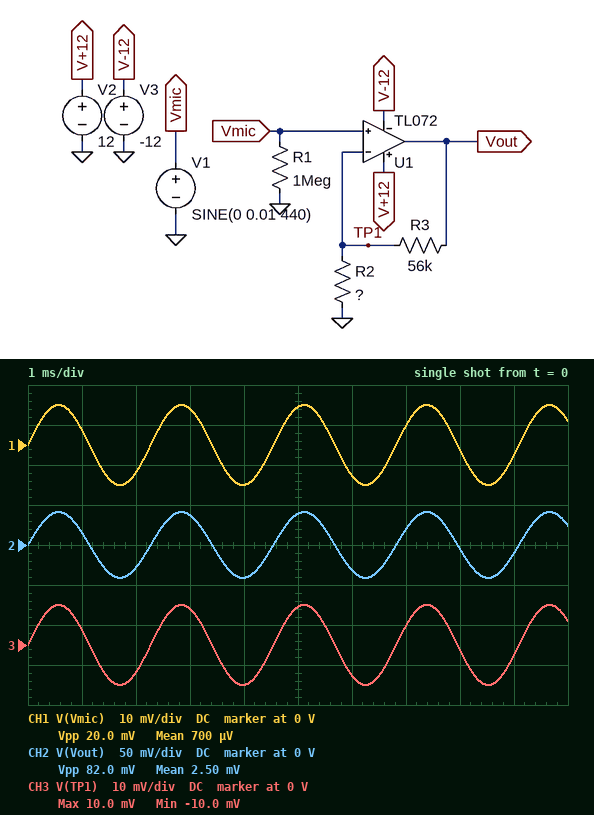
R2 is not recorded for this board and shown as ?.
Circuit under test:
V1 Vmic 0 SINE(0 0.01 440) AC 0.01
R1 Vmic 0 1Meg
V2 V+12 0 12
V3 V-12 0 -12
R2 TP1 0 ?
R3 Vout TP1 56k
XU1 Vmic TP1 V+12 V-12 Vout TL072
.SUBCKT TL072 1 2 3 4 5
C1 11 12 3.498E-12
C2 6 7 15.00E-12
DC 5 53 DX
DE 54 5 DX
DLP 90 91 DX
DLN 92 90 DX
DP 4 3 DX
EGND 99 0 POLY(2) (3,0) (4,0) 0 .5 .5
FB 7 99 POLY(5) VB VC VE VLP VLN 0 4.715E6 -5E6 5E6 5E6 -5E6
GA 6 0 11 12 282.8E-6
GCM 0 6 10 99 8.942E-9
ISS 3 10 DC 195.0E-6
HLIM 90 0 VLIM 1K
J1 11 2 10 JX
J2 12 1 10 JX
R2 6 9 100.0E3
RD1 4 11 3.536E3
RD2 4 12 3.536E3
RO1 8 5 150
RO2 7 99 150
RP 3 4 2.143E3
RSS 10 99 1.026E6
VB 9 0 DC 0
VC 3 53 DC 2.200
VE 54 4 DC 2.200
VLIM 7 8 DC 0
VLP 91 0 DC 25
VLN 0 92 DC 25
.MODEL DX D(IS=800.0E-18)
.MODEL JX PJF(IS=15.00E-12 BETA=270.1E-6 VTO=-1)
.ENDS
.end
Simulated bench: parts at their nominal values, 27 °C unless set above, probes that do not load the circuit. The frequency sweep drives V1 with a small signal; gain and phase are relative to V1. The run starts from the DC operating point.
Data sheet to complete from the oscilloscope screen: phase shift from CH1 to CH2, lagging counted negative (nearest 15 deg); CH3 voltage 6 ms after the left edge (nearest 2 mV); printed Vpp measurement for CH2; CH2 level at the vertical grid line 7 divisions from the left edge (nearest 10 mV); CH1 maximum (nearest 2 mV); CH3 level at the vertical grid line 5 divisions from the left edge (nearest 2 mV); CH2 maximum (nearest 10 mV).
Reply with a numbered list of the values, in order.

1. 0 deg
2. -8 mV
3. 82.0 mV
4. 20 mV
5. 10 mV
6. 10 mV
7. 40 mV
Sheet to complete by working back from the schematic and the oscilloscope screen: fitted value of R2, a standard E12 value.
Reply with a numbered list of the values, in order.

1. 18 kΩ
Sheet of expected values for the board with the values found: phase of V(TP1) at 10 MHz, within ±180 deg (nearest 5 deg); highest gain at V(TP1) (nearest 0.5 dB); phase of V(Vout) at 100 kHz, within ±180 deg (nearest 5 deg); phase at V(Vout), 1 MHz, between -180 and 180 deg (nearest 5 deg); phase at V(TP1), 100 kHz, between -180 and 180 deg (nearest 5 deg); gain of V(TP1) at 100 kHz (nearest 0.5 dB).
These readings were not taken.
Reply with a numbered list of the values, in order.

1. -145 deg
2. 0 dB
3. -5 deg
4. -55 deg
5. -5 deg
6. 0 dB
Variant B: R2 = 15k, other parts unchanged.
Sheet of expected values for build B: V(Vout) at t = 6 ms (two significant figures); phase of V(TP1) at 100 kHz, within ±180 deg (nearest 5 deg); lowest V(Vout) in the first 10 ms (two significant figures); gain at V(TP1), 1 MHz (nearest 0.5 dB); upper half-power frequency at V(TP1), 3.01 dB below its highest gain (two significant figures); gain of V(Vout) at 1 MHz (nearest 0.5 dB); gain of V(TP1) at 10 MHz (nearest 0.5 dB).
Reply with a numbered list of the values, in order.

1. -36 mV
2. -10 deg
3. -47 mV
4. -4.0 dB
5. 820 kHz
6. 9.5 dB
7. -28.0 dB
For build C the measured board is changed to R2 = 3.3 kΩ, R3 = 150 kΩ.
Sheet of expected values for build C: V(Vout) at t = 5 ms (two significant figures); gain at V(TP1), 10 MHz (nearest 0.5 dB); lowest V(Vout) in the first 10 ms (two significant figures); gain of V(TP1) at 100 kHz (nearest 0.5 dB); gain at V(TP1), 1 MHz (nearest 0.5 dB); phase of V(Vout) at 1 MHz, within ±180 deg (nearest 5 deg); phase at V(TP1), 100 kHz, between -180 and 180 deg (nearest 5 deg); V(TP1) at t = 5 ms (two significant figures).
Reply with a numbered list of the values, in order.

1. 440 mV
2. -48.0 dB
3. -460 mV
4. -4.5 dB
5. -22.5 dB
6. -95 deg
7. -55 deg
8. 9.5 mV
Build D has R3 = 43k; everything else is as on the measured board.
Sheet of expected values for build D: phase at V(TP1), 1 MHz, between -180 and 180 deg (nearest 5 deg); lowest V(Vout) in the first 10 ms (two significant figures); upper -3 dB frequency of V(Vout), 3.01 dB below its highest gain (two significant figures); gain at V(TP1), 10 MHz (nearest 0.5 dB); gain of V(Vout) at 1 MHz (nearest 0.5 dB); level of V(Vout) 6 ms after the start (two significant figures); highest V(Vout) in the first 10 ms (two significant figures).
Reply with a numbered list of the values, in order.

1. -50 deg
2. -34 mV
3. 1.2 MHz
4. -25.0 dB
5. 8.5 dB
6. -26 mV
7. 34 mV
